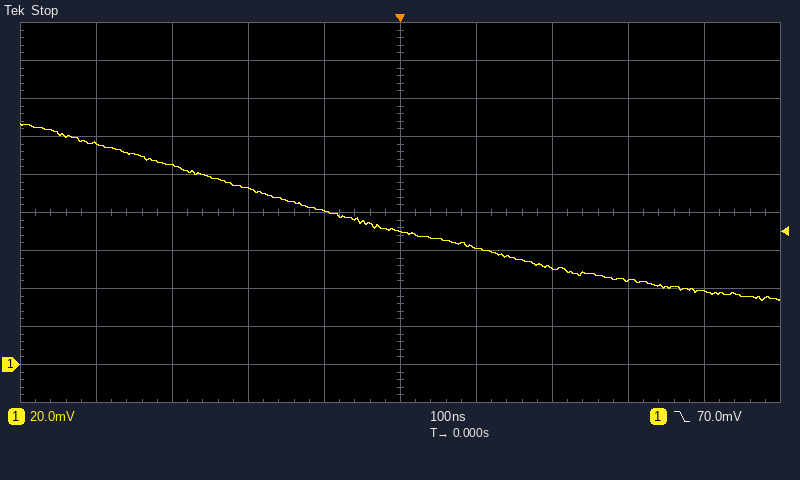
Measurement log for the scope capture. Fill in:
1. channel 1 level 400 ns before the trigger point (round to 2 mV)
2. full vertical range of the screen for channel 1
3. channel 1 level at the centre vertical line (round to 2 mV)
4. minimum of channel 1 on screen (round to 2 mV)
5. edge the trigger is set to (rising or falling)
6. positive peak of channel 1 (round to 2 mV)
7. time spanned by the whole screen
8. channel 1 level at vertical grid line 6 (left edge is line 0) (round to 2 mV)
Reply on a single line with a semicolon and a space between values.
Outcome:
116 mV; 200 mV; 70 mV; 34 mV; falling; 126 mV; 1 µs; 62 mV
